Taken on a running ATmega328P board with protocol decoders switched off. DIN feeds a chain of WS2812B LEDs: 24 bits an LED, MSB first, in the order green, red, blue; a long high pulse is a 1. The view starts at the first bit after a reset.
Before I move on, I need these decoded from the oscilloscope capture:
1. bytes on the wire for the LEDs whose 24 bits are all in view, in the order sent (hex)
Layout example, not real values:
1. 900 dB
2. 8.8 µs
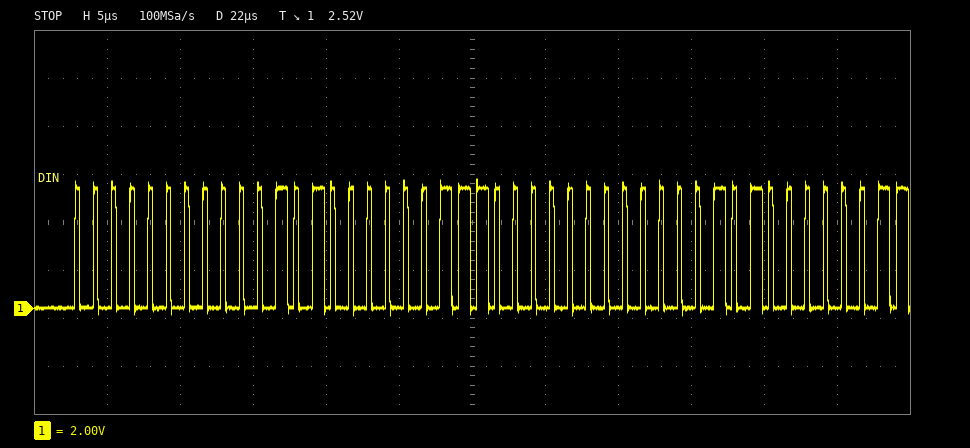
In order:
1. 00 14 0E
